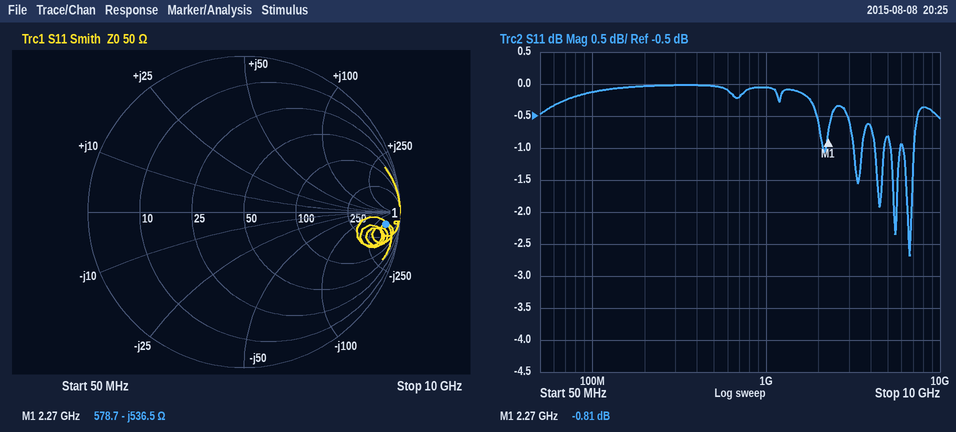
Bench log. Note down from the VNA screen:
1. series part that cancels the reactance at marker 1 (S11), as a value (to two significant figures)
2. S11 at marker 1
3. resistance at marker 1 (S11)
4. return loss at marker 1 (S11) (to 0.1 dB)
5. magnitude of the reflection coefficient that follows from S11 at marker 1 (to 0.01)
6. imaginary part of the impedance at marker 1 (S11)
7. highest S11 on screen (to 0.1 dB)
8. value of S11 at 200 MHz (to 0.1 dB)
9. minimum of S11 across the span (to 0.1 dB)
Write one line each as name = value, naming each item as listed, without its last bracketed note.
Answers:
series part that cancels the reactance at marker 1 (S11), as a value = 38 nH
S11 at marker 1 = -0.81 dB
resistance at marker 1 = 578.7 Ω
return loss at marker 1 (S11) = 0.8 dB
magnitude of the reflection coefficient that follows from S11 at marker 1 = 0.91
imaginary part of the impedance at marker 1 = -536.5 Ω
highest S11 on screen = 0.0 dB
value of S11 at 200 MHz = 0.0 dB
minimum of S11 across the span = -2.7 dB
